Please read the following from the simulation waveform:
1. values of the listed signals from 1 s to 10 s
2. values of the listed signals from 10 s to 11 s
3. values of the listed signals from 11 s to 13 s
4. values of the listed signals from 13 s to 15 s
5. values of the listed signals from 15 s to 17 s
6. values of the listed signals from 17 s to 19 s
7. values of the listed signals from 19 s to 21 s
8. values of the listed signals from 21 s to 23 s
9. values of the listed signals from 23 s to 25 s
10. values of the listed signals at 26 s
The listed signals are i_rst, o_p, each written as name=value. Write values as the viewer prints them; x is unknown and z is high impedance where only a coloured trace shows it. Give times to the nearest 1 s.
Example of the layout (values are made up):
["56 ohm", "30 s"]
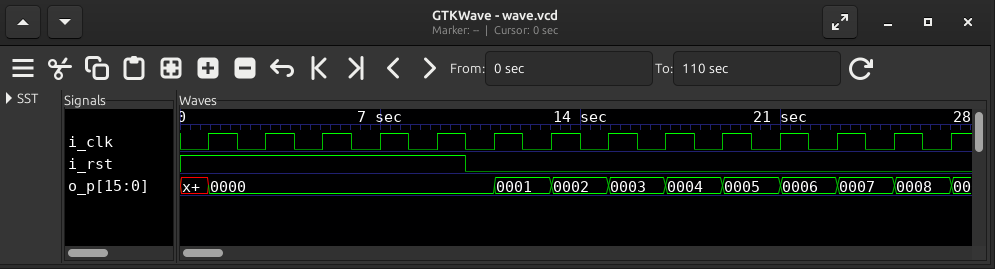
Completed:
["i_rst=1, o_p=0000", "i_rst=0, o_p=0000", "i_rst=0, o_p=0001", "i_rst=0, o_p=0002", "i_rst=0, o_p=0003", "i_rst=0, o_p=0004", "i_rst=0, o_p=0005", "i_rst=0, o_p=0006", "i_rst=0, o_p=0007", "i_rst=0, o_p=0008"]
